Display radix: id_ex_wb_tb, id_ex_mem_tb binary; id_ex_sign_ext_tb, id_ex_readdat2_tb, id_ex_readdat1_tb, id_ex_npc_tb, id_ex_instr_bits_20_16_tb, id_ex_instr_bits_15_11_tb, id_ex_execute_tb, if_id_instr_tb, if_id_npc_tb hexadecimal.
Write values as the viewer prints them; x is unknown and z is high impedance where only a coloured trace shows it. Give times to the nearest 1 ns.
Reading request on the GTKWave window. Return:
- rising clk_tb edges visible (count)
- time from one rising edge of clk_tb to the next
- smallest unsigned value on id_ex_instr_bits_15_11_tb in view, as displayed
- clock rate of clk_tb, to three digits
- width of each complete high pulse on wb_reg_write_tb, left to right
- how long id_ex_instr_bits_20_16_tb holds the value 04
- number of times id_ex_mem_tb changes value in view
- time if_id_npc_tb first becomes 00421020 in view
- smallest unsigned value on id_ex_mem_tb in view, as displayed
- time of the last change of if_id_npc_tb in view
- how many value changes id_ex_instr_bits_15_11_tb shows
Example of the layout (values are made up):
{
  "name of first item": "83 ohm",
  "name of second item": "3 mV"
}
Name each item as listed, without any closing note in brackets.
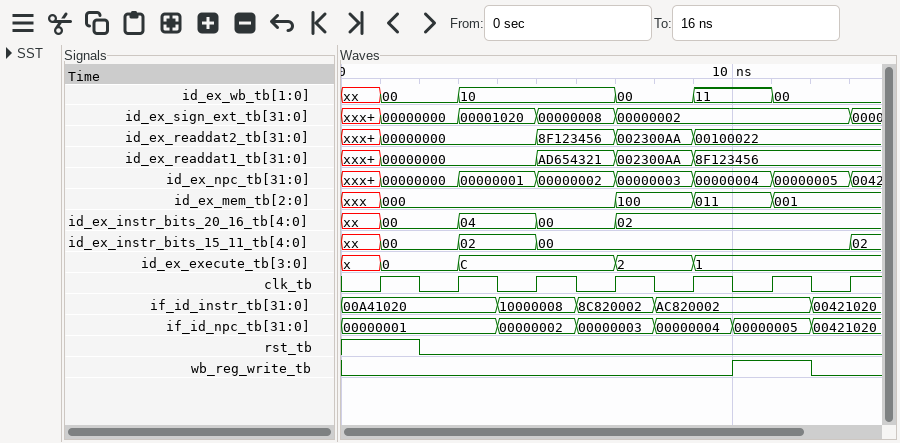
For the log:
{
  "rising clk_tb edges visible": "7",
  "time from one rising edge of clk_tb to the next": "2 ns",
  "smallest unsigned value on id_ex_instr_bits_15_11_tb in view, as displayed": "00",
  "clock rate of clk_tb, to three digits": "500 MHz",
  "width of each complete high pulse on wb_reg_write_tb, left to right": "2 ns",
  "how long id_ex_instr_bits_20_16_tb holds the value 04": "2 ns",
  "number of times id_ex_mem_tb changes value in view": "4",
  "time if_id_npc_tb first becomes 00421020 in view": "12 ns",
  "smallest unsigned value on id_ex_mem_tb in view, as displayed": "000",
  "time of the last change of if_id_npc_tb in view": "12 ns",
  "how many value changes id_ex_instr_bits_15_11_tb shows": "4"
}
